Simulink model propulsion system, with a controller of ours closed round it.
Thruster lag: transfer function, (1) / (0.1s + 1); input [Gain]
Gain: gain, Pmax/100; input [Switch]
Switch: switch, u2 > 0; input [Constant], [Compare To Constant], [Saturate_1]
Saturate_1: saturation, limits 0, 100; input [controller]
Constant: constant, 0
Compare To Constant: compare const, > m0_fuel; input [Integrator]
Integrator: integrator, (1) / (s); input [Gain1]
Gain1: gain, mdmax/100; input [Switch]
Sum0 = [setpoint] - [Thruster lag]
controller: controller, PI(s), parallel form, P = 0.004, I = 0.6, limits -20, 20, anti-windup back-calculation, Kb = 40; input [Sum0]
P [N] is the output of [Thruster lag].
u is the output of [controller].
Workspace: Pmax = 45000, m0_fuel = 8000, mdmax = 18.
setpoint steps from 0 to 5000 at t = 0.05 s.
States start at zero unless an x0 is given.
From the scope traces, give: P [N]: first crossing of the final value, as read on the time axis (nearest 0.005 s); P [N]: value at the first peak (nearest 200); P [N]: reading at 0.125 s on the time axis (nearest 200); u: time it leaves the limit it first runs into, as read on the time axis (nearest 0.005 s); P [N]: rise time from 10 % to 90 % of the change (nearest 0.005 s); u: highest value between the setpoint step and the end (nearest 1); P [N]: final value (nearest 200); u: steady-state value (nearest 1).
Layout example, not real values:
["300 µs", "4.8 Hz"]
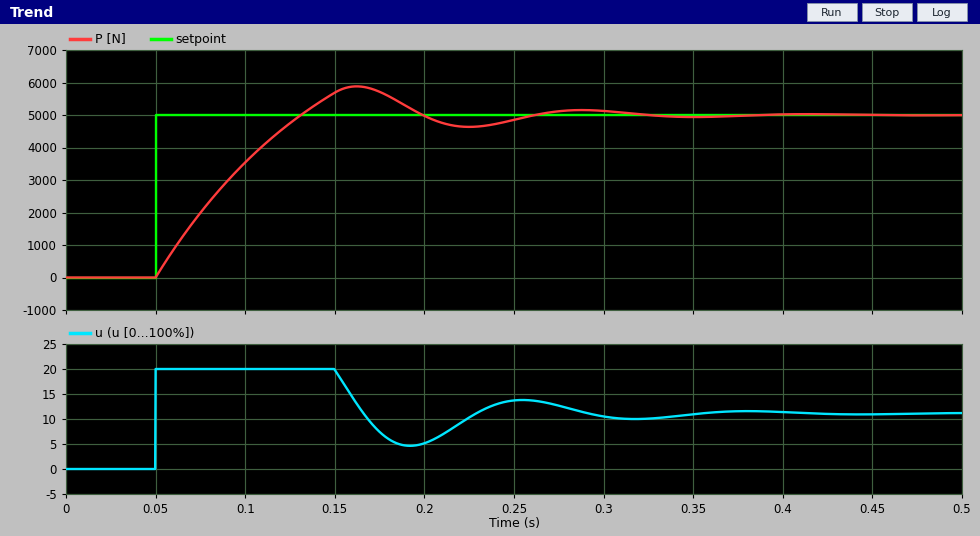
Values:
["0.130 s", "5800", "4800", "0.150 s", "0.065 s", "20", "5000", "11"]
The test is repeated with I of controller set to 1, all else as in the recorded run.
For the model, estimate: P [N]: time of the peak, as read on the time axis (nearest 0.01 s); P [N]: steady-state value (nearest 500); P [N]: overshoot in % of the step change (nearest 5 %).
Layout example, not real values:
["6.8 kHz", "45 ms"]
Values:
["0.16 s", "5000", "20 %"]
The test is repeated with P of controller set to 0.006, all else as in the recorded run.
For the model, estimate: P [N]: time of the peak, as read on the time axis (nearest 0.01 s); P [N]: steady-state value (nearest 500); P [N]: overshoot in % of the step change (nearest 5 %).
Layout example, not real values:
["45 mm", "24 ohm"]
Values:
["0.16 s", "5000", "15 %"]
